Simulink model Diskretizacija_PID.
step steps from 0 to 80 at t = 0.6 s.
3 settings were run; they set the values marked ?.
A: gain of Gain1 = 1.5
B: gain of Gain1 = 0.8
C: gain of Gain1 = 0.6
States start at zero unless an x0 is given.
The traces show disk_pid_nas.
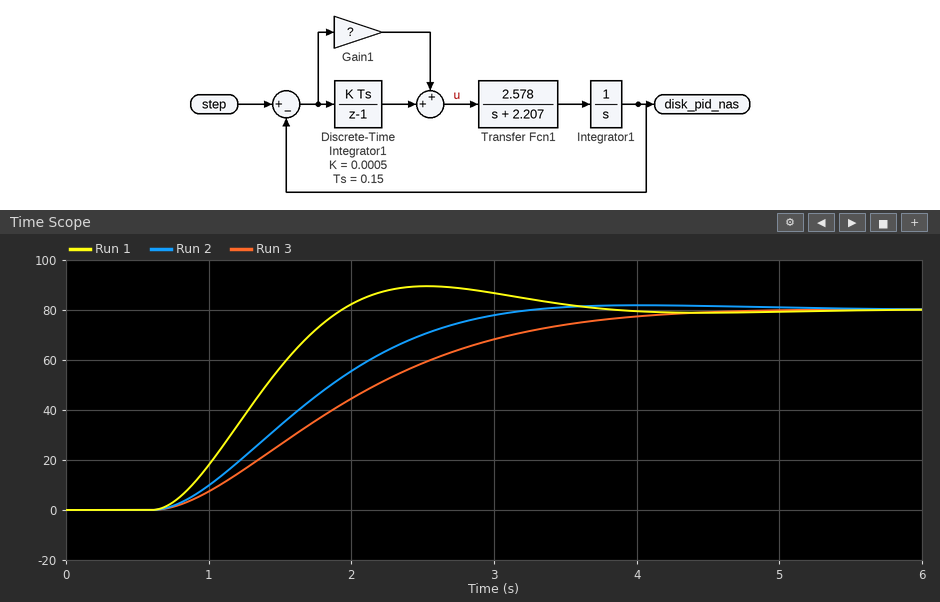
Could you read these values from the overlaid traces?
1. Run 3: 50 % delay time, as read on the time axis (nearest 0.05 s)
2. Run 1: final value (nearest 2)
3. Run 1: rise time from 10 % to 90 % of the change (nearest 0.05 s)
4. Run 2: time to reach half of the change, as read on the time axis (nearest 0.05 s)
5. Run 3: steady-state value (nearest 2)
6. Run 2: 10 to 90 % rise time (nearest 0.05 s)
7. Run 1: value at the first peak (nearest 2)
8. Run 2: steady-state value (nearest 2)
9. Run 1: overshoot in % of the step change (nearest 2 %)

1.85 s
80
0.90 s
1.65 s
80
1.65 s
90
80
12 %
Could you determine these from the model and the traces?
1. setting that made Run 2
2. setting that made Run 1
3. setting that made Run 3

B
A
C
